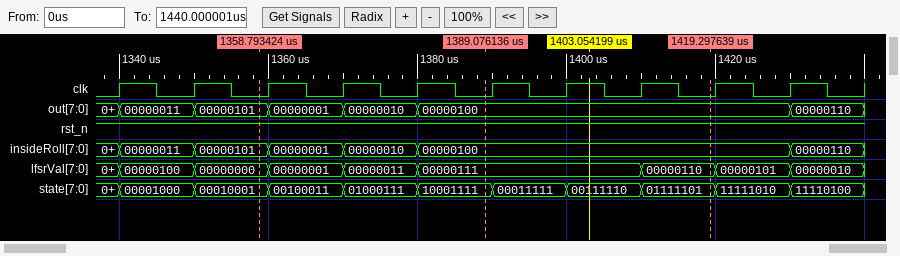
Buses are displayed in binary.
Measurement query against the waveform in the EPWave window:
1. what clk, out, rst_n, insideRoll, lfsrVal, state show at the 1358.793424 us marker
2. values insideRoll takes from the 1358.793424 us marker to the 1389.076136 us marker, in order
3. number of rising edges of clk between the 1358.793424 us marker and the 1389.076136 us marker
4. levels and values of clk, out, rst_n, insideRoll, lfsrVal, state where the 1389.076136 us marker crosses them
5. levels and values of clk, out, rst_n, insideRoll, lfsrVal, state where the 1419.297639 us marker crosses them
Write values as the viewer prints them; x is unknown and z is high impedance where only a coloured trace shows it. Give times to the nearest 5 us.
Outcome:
clk=0, out=00000101, rst_n=1, insideRoll=00000101, lfsrVal=00000000, state=00010001
00000101, 00000001, 00000010, 00000100
3
clk=0, out=00000100, rst_n=1, insideRoll=00000100, lfsrVal=00000111, state=10001111
clk=0, out=00000100, rst_n=1, insideRoll=00000100, lfsrVal=00000110, state=01111101
